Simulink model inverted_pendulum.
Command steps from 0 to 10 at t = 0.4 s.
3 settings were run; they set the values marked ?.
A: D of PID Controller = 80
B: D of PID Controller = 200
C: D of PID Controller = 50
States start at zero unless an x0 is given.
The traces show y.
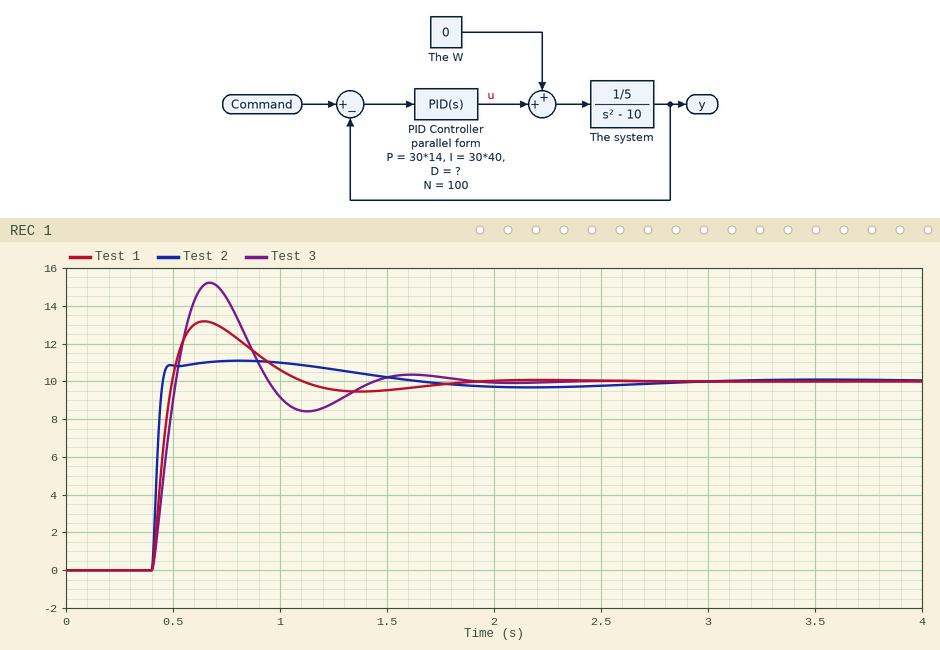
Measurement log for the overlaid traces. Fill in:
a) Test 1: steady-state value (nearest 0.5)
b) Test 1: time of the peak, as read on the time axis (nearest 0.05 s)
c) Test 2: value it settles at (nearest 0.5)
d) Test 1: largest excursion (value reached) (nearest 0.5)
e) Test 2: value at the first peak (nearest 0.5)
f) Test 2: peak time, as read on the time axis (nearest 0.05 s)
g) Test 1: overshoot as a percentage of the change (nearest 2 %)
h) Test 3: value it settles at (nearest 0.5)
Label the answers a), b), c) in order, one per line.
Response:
a) 10.0
b) 0.65 s
c) 10.0
d) 13.0
e) 11.0
f) 0.80 s
g) 32 %
h) 10.0
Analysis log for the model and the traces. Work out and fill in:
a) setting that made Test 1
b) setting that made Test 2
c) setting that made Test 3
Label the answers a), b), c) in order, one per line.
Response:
a) A
b) B
c) C
